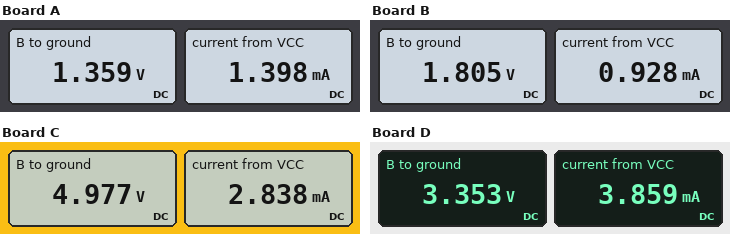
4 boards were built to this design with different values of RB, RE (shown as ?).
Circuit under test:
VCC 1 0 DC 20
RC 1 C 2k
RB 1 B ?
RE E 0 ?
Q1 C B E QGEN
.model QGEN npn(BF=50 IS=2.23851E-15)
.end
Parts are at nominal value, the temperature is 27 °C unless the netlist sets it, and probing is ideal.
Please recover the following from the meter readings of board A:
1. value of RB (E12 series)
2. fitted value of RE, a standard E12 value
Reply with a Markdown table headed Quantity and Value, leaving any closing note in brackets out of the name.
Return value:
| Quantity | Value |
|---|---|
| value of RB | 680 kΩ |
| fitted value of RE, a standard E12 value | 470 Ω |
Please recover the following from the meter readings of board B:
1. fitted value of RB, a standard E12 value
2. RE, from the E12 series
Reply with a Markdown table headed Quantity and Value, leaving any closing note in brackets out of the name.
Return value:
| Quantity | Value |
|---|---|
| fitted value of RB, a standard E12 value | 1 MΩ |
| RE, from the E12 series | 1.2 kΩ |
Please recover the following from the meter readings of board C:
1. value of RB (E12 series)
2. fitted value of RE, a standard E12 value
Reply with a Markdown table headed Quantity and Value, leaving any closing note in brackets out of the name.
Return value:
| Quantity | Value |
|---|---|
| value of RB | 270 kΩ |
| fitted value of RE, a standard E12 value | 1.5 kΩ |
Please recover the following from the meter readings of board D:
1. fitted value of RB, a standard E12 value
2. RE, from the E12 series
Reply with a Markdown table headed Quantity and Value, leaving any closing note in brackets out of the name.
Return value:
| Quantity | Value |
|---|---|
| fitted value of RB, a standard E12 value | 220 kΩ |
| RE, from the E12 series | 680 Ω |
